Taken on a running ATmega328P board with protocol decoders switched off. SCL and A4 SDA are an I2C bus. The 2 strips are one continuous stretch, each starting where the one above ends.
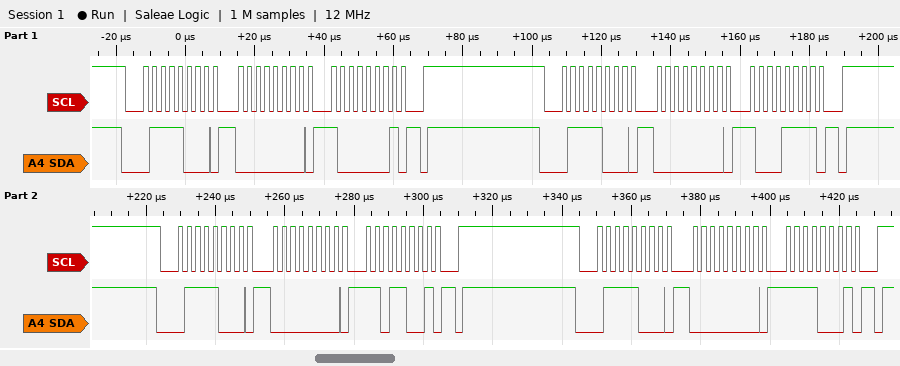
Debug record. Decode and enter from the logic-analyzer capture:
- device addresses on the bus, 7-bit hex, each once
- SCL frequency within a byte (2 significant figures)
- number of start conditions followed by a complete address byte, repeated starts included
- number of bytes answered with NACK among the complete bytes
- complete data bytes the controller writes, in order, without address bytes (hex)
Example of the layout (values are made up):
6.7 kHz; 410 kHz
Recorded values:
0x3C; 400 kHz; 4; 0; 00 81 00 8F 00 D9 00 F1
